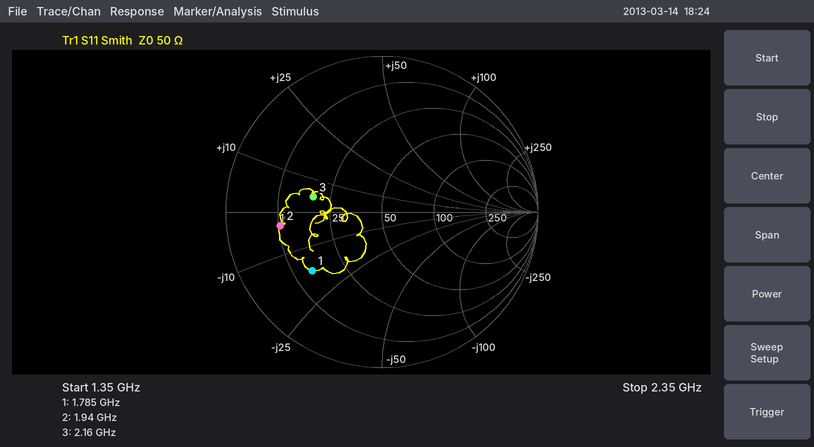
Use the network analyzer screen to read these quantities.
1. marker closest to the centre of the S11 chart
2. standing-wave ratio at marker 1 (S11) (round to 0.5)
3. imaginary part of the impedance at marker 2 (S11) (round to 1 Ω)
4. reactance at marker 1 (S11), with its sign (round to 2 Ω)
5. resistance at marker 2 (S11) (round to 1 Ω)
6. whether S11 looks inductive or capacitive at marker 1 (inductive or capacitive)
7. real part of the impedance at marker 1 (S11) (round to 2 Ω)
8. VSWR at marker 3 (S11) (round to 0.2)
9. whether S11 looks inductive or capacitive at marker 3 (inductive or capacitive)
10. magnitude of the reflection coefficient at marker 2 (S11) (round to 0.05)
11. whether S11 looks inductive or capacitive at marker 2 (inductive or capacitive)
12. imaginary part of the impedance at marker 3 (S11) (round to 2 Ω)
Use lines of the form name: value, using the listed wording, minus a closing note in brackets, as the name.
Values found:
marker closest to the centre of the S11 chart: marker 3
standing-wave ratio at marker 1 (S11): 4.0
imaginary part of the impedance at marker 2 (S11): -3 Ω
reactance at marker 1 (S11), with its sign: -16 Ω
resistance at marker 2 (S11): 10 Ω
whether S11 looks inductive or capacitive at marker 1: capacitive
real part of the impedance at marker 1 (S11): 14 Ω
VSWR at marker 3 (S11): 2.6
whether S11 looks inductive or capacitive at marker 3: inductive
magnitude of the reflection coefficient at marker 2 (S11): 0.65
whether S11 looks inductive or capacitive at marker 2: capacitive
imaginary part of the impedance at marker 3 (S11): +4 Ω
